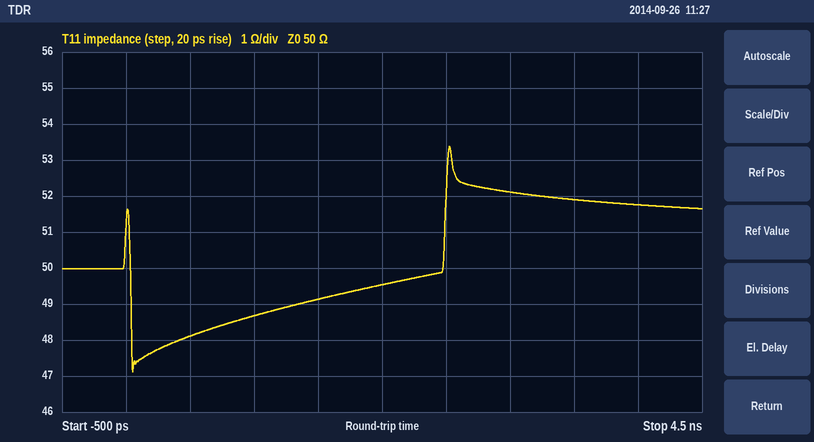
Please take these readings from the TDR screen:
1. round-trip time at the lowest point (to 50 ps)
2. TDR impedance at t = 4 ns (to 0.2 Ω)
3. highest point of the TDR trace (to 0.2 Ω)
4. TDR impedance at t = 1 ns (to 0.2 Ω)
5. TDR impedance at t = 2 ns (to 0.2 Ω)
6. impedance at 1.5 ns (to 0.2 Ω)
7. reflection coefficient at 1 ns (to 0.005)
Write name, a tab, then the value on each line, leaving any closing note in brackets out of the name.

round-trip time at the lowest point	50 ps
TDR impedance at t = 4 ns	51.8 Ω
highest point of the TDR trace	53.4 Ω
TDR impedance at t = 1 ns	48.6 Ω
TDR impedance at t = 2 ns	49.6 Ω
impedance at 1.5 ns	49.2 Ω
reflection coefficient at 1 ns	-0.015
